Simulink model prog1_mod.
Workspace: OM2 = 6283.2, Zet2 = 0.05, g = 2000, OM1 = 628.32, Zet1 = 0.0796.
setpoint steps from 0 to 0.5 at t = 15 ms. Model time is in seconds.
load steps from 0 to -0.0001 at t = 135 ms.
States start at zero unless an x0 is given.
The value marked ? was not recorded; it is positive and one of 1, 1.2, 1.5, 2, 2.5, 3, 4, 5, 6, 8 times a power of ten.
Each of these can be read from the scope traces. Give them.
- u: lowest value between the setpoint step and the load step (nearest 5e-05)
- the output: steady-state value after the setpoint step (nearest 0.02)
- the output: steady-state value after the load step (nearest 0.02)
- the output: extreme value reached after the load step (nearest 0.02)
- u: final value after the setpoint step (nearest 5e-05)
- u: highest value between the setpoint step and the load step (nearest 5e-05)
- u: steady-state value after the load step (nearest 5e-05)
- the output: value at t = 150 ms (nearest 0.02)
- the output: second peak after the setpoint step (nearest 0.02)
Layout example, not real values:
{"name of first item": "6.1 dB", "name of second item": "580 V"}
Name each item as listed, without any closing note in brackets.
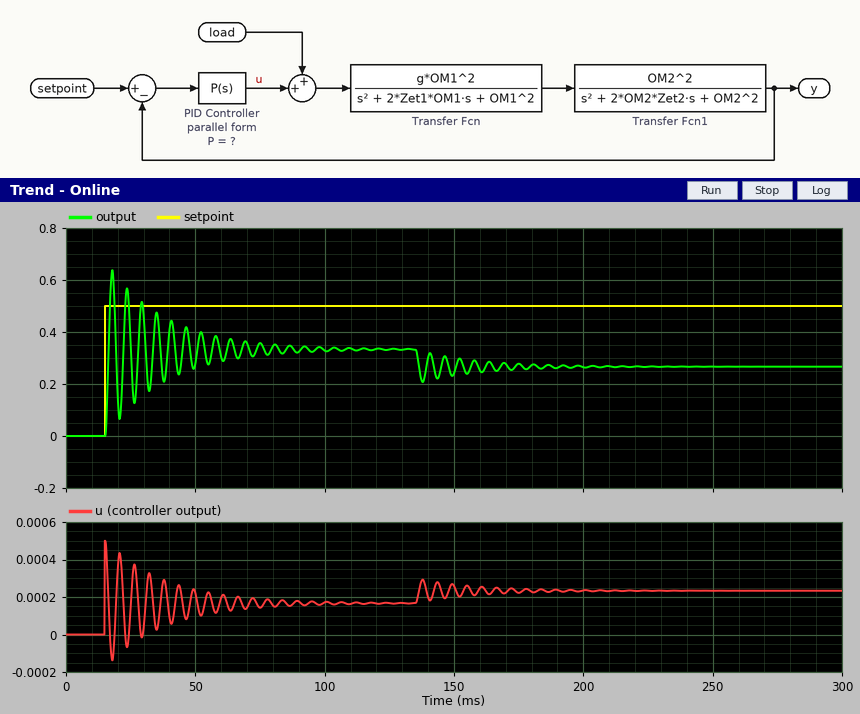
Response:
{"u: lowest value between the setpoint step and the load step": "-0.00015", "the output: steady-state value after the setpoint step": "0.34", "the output: steady-state value after the load step": "0.26", "the output: extreme value reached after the load step": "0.20", "u: final value after the setpoint step": "0.00015", "u: highest value between the setpoint step and the load step": "0.00050", "u: steady-state value after the load step": "0.00025", "the output: value at t = 150 ms": "0.24", "the output: second peak after the setpoint step": "0.56"}
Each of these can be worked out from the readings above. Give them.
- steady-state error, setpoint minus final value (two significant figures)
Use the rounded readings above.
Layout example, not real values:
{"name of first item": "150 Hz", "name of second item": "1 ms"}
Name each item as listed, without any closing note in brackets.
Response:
{"steady-state error, setpoint minus final value": "0.16"}
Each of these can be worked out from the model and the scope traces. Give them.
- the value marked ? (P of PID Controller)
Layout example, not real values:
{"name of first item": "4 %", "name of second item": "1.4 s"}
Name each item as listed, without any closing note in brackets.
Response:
{"the value marked ?": "0.001"}
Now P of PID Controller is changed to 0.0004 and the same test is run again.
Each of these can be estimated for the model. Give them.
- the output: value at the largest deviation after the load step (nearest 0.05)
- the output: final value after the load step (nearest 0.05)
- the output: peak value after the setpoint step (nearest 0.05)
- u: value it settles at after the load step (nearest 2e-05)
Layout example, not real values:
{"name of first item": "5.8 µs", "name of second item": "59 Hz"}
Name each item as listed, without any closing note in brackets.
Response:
{"the output: value at the largest deviation after the load step": "0.00", "the output: final value after the load step": "0.10", "the output: peak value after the setpoint step": "0.40", "u: value it settles at after the load step": "0.00016"}
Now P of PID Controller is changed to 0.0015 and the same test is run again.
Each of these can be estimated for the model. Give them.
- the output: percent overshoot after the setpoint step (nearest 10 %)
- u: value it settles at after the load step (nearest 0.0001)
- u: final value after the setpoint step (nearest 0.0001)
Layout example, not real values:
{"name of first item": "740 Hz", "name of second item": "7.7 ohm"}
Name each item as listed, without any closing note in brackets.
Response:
{"the output: percent overshoot after the setpoint step": "90 %", "u: value it settles at after the load step": "0.0003", "u: final value after the setpoint step": "0.0002"}
